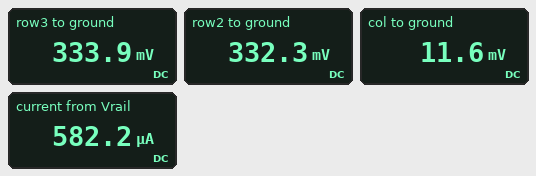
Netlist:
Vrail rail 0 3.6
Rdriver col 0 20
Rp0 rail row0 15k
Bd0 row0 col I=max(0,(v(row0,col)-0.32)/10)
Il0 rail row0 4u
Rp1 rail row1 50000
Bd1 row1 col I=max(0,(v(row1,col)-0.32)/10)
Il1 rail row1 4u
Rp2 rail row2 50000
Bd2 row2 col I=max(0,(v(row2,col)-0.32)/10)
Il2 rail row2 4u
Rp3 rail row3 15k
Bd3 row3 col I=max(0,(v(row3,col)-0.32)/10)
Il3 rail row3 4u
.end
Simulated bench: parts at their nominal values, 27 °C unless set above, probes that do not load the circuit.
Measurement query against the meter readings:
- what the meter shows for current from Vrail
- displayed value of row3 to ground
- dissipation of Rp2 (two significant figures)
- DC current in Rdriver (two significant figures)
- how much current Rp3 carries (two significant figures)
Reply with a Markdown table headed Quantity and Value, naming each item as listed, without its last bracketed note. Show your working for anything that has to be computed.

| Quantity | Value |
|---|---|
| what the meter shows for current from Vrail | 582.2 µA |
| displayed value of row3 to ground | 333.9 mV |
| dissipation of Rp2 | (3.6 V - 332.3 mV)^2 / 50 kΩ = 210 µW |
| DC current in Rdriver | (11.6 mV) / 20 Ω = 580 µA |
| how much current Rp3 carries | (3.6 V - 333.9 mV) / 15 kΩ = 220 µA |
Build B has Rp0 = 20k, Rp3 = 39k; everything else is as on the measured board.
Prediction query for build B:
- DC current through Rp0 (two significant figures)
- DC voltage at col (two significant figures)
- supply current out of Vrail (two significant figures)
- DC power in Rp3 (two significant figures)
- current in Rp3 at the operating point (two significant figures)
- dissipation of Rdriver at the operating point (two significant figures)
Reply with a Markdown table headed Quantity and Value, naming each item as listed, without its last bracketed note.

| Quantity | Value |
|---|---|
| DC current through Rp0 | 160 µA |
| DC voltage at col | 7.9 mV |
| supply current out of Vrail | 390 µA |
| DC power in Rp3 | 270 µW |
| current in Rp3 at the operating point | 84 µA |
| dissipation of Rdriver at the operating point | 3.1 µW |
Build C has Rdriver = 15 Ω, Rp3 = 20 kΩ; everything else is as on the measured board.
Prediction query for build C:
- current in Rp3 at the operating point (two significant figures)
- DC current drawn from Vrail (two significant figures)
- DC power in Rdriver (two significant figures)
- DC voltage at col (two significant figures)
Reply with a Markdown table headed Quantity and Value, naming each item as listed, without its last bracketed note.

| Quantity | Value |
|---|---|
| current in Rp3 at the operating point | 160 µA |
| DC current drawn from Vrail | 530 µA |
| DC power in Rdriver | 4.2 µW |
| DC voltage at col | 7.9 mV |
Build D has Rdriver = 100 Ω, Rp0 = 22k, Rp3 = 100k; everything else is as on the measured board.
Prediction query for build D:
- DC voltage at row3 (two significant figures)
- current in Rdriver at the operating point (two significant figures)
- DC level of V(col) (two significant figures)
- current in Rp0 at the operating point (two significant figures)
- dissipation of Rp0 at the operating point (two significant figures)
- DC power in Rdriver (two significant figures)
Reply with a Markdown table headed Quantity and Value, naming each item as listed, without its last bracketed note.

| Quantity | Value |
|---|---|
| DC voltage at row3 | 350 mV |
| current in Rdriver at the operating point | 330 µA |
| DC level of V(col) | 33 mV |
| current in Rp0 at the operating point | 150 µA |
| dissipation of Rp0 at the operating point | 480 µW |
| DC power in Rdriver | 11 µW |
